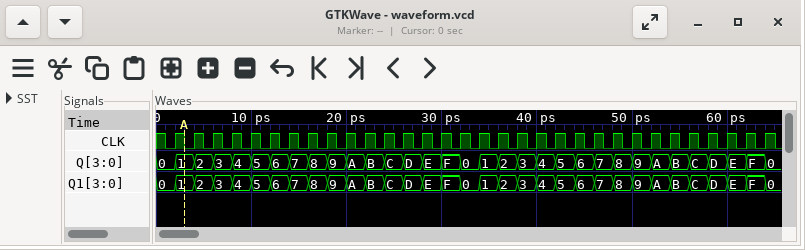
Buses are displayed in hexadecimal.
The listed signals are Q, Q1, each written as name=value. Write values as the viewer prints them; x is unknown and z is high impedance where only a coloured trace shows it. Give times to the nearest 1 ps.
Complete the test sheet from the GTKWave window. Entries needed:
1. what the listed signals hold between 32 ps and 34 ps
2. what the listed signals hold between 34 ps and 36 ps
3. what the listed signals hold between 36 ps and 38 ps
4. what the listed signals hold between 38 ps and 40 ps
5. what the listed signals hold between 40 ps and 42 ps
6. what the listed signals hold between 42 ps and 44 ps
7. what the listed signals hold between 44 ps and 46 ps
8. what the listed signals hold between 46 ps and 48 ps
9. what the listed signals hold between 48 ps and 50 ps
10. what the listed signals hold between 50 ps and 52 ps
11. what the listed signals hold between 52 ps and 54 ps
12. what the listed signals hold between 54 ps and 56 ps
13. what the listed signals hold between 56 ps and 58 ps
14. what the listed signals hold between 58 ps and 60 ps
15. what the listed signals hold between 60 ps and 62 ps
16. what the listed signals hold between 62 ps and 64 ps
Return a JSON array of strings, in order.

["Q=0, Q1=0", "Q=1, Q1=1", "Q=2, Q1=2", "Q=3, Q1=3", "Q=4, Q1=4", "Q=5, Q1=5", "Q=6, Q1=6", "Q=7, Q1=7", "Q=8, Q1=8", "Q=9, Q1=9", "Q=A, Q1=A", "Q=B, Q1=B", "Q=C, Q1=C", "Q=D, Q1=D", "Q=E, Q1=E", "Q=F, Q1=F"]
